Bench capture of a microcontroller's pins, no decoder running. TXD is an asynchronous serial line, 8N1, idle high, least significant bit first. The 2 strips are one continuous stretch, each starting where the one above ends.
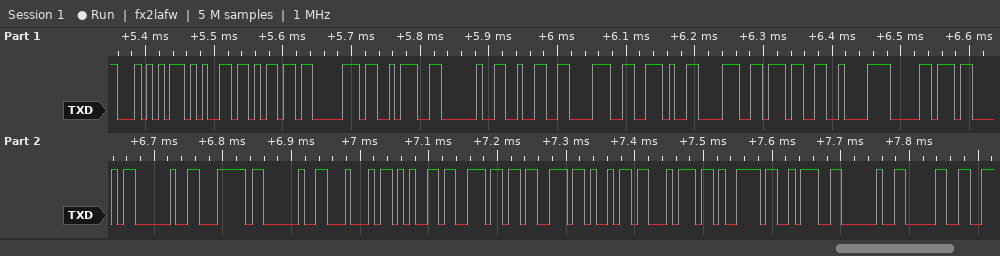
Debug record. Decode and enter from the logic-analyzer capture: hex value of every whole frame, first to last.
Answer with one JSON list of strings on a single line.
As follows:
["54 65 6D 70 3A 20 32 38 2E 38 37 C2 B0 43 20 7C 20 44 65 6E 73 69 74 79 3A 20 30"]
